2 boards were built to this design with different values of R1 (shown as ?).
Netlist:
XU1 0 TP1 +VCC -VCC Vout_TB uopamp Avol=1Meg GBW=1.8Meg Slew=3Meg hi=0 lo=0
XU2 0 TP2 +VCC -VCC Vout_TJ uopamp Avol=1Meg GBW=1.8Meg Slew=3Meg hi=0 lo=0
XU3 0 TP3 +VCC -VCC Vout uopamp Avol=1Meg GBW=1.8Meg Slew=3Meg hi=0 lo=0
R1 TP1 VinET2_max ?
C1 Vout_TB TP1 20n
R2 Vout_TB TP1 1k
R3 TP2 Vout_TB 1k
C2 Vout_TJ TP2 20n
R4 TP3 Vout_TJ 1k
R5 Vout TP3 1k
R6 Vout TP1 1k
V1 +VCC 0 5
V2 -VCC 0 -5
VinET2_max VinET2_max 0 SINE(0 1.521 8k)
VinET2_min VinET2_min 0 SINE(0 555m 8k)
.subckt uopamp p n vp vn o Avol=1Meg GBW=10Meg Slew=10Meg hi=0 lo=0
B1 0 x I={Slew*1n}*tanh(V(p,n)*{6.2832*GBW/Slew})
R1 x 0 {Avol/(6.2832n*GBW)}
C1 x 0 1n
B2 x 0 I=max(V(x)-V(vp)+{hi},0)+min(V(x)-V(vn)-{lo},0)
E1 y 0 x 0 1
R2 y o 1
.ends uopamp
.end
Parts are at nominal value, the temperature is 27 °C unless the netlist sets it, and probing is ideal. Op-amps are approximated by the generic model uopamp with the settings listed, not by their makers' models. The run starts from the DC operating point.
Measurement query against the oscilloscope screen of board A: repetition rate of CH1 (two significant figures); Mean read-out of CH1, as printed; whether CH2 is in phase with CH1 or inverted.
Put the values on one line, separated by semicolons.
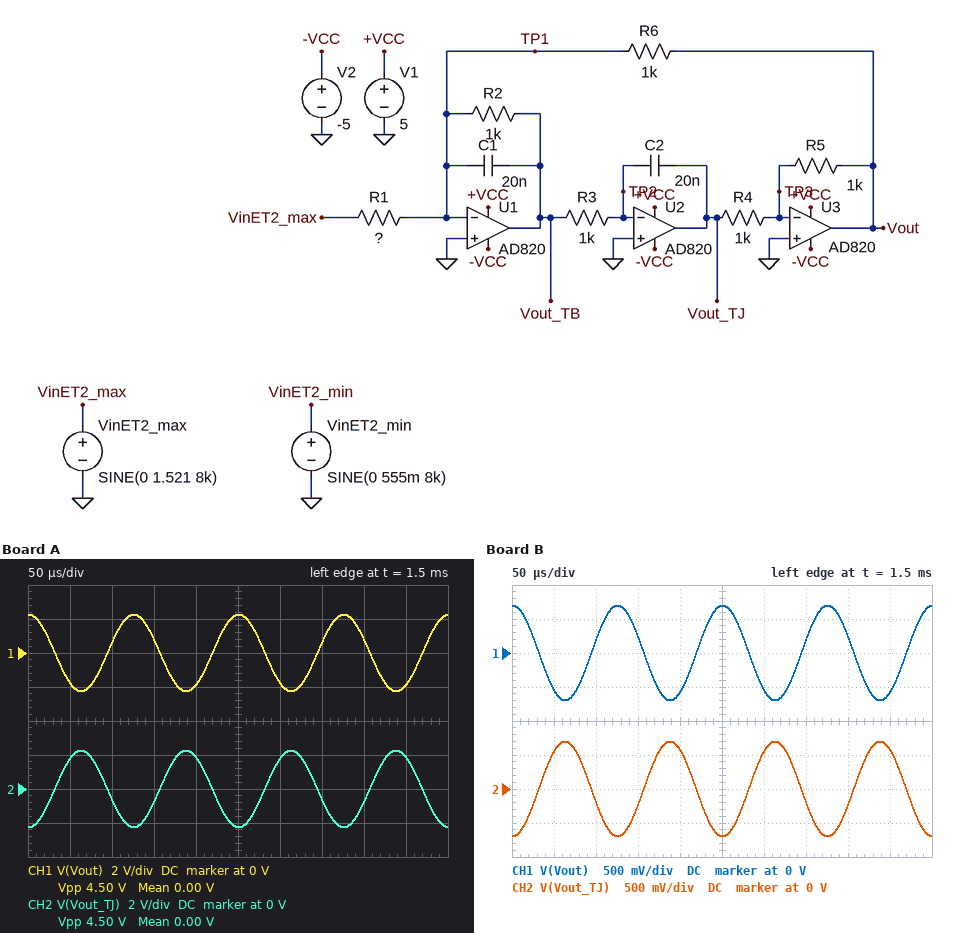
8.0 kHz; 0.00 V; inverted
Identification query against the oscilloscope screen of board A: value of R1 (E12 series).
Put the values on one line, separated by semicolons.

680 Ω
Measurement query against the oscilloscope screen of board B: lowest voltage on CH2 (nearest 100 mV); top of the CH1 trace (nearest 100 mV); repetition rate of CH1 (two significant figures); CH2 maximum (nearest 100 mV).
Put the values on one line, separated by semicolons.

-700 mV; 700 mV; 8.0 kHz; 700 mV
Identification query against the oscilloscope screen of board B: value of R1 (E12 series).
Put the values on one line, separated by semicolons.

2.2 kΩ
